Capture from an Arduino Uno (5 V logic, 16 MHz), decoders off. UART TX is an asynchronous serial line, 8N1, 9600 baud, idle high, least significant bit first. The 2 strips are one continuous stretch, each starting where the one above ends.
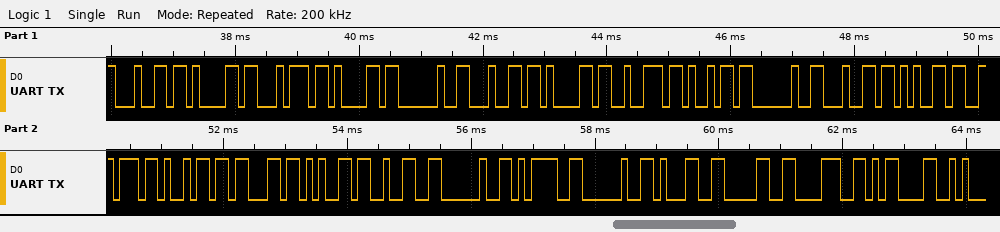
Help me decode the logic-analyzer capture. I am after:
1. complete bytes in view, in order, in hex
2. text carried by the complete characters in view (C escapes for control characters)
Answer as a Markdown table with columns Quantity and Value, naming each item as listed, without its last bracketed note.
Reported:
| Quantity | Value |
|---|---|
| complete bytes in view, in order, in hex | 64 61 74 61 20 64 61 72 69 20 64 65 76 69 63 65 32 20 3D 20 31 30 38 0D |
| text carried by the complete characters in view | "data dari device2 = 108\r" |
